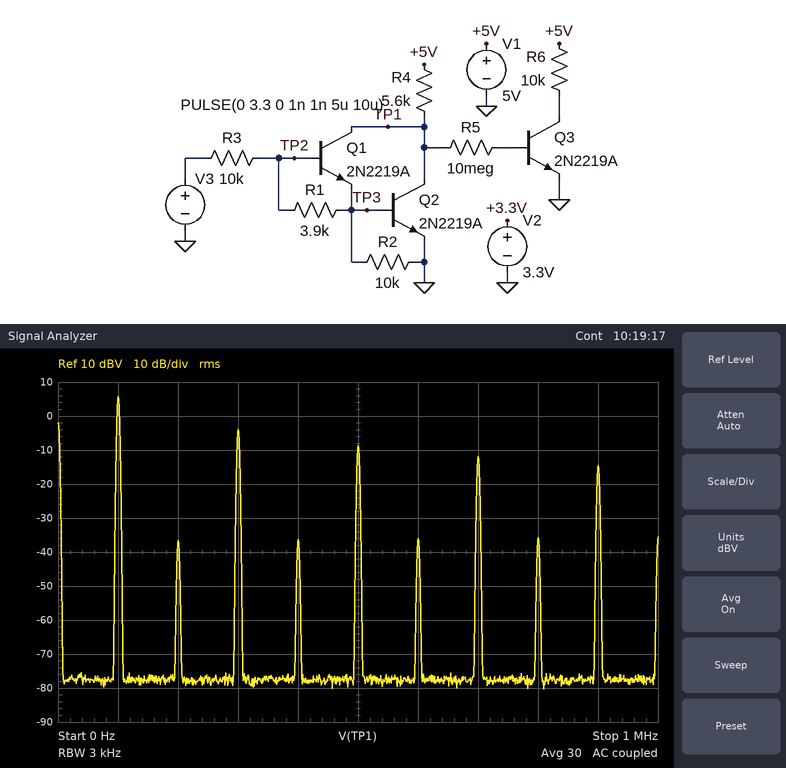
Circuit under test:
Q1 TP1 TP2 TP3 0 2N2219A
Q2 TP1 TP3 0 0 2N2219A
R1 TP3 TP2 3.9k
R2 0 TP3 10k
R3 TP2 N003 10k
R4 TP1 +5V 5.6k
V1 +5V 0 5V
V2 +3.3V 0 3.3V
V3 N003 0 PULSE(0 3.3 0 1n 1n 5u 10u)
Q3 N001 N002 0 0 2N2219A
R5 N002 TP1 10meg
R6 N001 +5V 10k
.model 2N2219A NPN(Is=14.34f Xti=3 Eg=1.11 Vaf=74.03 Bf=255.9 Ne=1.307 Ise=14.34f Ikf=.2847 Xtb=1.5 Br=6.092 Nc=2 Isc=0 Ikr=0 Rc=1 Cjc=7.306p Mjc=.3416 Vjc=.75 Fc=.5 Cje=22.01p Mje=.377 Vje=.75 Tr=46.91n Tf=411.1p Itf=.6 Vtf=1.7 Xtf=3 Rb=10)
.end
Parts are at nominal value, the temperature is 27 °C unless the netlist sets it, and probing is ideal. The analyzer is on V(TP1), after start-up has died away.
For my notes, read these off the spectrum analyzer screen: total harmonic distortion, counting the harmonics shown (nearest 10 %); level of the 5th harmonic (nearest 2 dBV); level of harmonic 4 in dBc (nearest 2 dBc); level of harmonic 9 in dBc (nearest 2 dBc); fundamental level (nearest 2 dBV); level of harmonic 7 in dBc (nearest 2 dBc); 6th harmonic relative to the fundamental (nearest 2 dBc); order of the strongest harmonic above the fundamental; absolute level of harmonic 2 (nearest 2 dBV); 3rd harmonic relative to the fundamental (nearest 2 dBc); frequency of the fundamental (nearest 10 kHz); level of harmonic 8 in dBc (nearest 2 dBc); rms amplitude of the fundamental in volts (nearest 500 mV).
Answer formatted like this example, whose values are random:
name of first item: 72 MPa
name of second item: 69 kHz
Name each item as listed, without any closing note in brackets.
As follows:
total harmonic distortion, counting the harmonics shown: 40 %
level of the 5th harmonic: -8 dBV
level of harmonic 4 in dBc: -42 dBc
level of harmonic 9 in dBc: -20 dBc
fundamental level: 6 dBV
level of harmonic 7 in dBc: -18 dBc
6th harmonic relative to the fundamental: -42 dBc
order of the strongest harmonic above the fundamental: 3
absolute level of harmonic 2: -36 dBV
3rd harmonic relative to the fundamental: -10 dBc
frequency of the fundamental: 100 kHz
level of harmonic 8 in dBc: -42 dBc
rms amplitude of the fundamental in volts: 2.0 V
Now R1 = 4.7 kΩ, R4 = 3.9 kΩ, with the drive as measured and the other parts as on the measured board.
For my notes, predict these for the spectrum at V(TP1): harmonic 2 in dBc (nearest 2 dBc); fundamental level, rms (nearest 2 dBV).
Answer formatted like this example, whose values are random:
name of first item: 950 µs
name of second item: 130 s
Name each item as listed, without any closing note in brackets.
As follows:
harmonic 2 in dBc: -36 dBc
fundamental level, rms: 6 dBV
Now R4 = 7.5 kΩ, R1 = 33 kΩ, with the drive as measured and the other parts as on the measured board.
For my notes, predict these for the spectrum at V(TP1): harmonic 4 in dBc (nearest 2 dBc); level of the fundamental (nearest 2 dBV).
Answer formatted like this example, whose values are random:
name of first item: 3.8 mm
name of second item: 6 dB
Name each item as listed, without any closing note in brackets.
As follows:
harmonic 4 in dBc: -22 dBc
level of the fundamental: 6 dBV
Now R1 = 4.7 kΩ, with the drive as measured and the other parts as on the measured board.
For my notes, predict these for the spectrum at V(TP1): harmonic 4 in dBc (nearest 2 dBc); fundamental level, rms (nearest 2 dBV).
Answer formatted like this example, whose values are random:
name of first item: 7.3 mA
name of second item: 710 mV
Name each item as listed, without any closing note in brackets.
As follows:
harmonic 4 in dBc: -36 dBc
fundamental level, rms: 6 dBV
